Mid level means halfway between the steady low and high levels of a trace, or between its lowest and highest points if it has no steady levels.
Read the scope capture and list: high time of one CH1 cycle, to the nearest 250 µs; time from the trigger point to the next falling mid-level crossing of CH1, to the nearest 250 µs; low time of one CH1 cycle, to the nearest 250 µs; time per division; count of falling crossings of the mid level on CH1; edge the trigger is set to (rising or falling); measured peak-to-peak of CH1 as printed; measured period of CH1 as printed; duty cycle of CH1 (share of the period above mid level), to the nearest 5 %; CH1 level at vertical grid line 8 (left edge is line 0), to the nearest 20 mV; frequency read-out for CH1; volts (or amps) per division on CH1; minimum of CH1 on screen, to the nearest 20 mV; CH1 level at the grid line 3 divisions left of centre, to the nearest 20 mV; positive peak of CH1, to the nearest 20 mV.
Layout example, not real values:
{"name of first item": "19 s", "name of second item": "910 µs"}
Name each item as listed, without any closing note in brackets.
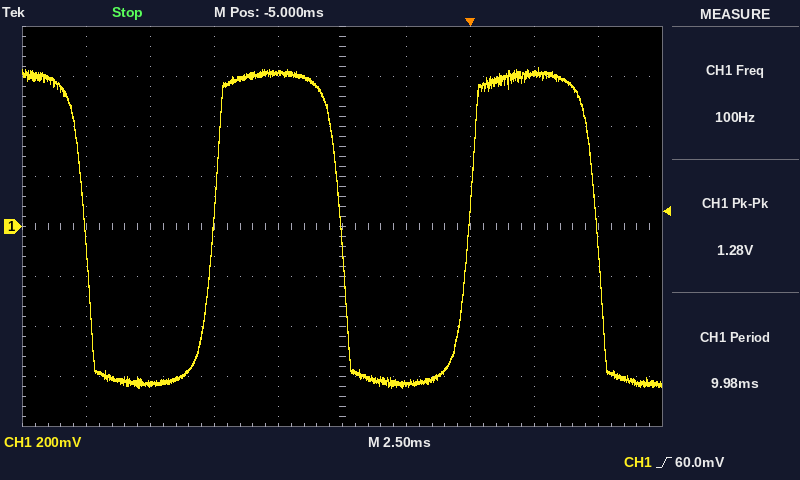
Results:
{"high time of one CH1 cycle, to the nearest 250 µs": "5.00 ms", "time from the trigger point to the next falling mid-level crossing of CH1, to the nearest 250 µs": "5.00 ms", "low time of one CH1 cycle, to the nearest 250 µs": "5.00 ms", "time per division": "2.5 ms", "count of falling crossings of the mid level on CH1": "3", "edge the trigger is set to": "rising", "measured peak-to-peak of CH1 as printed": "1.28 V", "measured period of CH1 as printed": "9.98 ms", "duty cycle of CH1 (share of the period above mid level), to the nearest 5 %": "50 %", "CH1 level at vertical grid line 8 (left edge is line 0), to the nearest 20 mV": "620 mV", "frequency read-out for CH1": "100 Hz", "volts (or amps) per division on CH1": "200 mV", "minimum of CH1 on screen, to the nearest 20 mV": "-640 mV", "CH1 level at the grid line 3 divisions left of centre, to the nearest 20 mV": "-620 mV", "positive peak of CH1, to the nearest 20 mV": "640 mV"}
